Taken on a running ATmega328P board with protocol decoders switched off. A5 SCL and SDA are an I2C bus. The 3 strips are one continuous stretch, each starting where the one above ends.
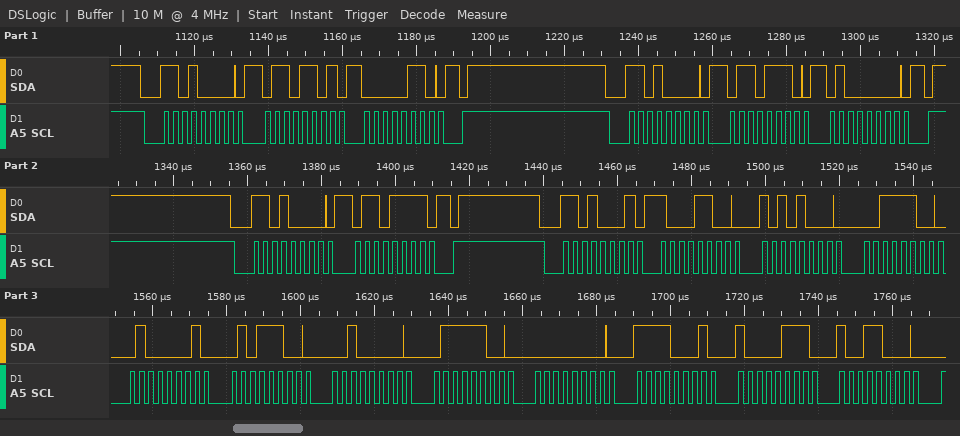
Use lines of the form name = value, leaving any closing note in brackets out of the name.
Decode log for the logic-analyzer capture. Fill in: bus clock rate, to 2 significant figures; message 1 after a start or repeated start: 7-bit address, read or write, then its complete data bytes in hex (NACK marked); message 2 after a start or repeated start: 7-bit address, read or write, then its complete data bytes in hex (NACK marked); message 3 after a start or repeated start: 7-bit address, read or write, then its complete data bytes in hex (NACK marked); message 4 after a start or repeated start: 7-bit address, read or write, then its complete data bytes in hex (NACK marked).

bus clock rate, to 2 significant figures = 400 kHz
message 1 after a start or repeated start: 7-bit address, read or write, then its complete data bytes in hex = 0x68 write: 6D 06
message 2 after a start or repeated start: 7-bit address, read or write, then its complete data bytes in hex = 0x68 write: 6E 40
message 3 after a start or repeated start: 7-bit address, read or write, then its complete data bytes in hex = 0x68 write: 6F
message 4 after a start or repeated start: 7-bit address, read or write, then its complete data bytes in hex = 0x68 read: 8C A8 3C 41 5C 20 7C 00 F1 87 98
